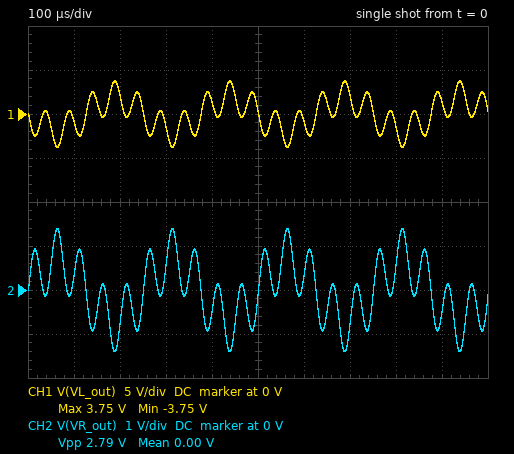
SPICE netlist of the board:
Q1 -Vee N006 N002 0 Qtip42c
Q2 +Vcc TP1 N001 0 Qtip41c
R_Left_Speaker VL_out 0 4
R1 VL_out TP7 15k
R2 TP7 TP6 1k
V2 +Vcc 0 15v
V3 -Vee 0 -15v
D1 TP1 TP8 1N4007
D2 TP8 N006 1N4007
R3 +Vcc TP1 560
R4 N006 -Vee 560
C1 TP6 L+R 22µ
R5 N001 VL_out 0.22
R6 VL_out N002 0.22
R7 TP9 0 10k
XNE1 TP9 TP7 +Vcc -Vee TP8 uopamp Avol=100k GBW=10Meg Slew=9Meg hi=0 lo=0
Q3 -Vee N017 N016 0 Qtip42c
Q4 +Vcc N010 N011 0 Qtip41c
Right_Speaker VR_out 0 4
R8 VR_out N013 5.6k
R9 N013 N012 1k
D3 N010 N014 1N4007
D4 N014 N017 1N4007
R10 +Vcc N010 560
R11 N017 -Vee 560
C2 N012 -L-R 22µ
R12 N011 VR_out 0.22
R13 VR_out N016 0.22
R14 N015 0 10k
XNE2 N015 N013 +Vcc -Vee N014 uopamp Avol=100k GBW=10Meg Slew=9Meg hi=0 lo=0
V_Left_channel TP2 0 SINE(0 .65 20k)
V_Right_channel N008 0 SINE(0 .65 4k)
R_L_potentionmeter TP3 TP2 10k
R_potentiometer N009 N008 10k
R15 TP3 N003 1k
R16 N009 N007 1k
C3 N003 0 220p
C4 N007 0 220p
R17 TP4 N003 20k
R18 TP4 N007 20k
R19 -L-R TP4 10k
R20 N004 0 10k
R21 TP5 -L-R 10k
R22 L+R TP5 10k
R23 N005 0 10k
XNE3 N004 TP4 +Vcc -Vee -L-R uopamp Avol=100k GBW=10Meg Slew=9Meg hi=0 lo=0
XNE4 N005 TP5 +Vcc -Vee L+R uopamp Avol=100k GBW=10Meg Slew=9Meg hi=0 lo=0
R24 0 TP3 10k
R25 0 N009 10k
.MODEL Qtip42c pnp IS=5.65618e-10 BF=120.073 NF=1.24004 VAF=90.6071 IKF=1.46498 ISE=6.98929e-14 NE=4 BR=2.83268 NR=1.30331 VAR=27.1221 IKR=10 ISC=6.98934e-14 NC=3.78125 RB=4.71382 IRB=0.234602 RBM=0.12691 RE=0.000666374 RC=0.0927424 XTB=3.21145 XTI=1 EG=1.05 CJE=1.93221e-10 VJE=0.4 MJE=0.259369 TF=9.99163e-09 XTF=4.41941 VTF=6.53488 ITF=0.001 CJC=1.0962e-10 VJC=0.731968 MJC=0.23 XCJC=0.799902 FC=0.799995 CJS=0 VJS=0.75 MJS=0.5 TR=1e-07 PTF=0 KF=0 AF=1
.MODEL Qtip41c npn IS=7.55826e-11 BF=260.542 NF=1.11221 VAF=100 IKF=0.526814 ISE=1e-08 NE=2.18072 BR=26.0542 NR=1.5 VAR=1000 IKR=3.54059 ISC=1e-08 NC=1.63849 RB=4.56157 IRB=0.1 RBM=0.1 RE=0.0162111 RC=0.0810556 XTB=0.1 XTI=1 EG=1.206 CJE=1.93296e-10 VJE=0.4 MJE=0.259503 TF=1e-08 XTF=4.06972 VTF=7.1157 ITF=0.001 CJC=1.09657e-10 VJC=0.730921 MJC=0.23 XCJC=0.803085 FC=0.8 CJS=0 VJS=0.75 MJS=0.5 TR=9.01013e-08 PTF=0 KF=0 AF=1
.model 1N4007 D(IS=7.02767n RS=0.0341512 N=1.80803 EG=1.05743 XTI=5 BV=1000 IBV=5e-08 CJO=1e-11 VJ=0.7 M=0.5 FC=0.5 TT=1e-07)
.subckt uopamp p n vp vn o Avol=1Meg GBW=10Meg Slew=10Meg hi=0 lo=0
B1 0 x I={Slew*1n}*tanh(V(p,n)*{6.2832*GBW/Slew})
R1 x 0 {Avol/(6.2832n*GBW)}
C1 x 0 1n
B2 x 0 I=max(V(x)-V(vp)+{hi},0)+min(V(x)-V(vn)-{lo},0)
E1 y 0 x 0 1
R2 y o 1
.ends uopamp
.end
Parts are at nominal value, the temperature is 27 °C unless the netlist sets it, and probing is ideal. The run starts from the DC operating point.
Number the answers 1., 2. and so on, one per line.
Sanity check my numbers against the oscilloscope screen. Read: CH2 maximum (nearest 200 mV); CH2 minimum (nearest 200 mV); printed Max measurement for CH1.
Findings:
1. 1.4 V
2. -1.4 V
3. 3.75 V
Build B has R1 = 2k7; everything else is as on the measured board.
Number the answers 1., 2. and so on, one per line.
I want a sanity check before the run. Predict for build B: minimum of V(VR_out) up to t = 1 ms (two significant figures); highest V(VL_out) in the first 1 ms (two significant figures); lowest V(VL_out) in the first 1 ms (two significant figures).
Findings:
1. -1.4 V
2. 670 mV
3. -670 mV
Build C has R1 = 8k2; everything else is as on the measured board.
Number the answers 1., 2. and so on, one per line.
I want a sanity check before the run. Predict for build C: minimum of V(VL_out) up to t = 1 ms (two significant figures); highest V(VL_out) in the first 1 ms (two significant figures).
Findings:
1. -2.0 V
2. 2.0 V
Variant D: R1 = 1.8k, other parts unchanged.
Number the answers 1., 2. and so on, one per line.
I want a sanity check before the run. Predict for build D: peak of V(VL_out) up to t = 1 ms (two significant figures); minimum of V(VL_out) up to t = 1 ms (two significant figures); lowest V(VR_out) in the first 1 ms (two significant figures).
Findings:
1. 450 mV
2. -450 mV
3. -1.4 V
